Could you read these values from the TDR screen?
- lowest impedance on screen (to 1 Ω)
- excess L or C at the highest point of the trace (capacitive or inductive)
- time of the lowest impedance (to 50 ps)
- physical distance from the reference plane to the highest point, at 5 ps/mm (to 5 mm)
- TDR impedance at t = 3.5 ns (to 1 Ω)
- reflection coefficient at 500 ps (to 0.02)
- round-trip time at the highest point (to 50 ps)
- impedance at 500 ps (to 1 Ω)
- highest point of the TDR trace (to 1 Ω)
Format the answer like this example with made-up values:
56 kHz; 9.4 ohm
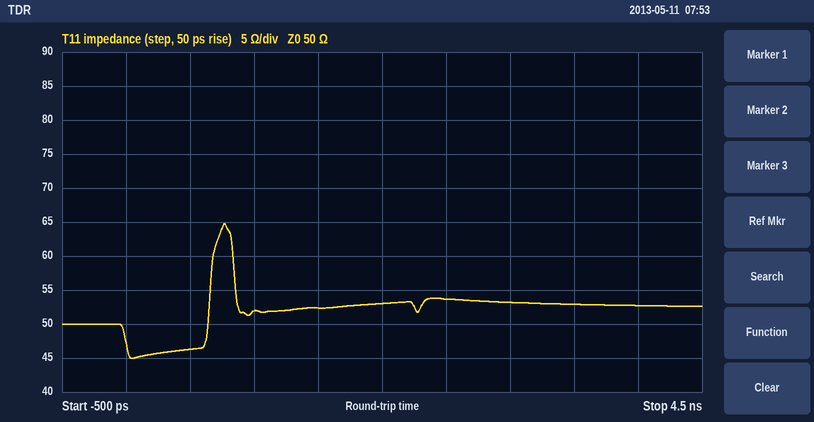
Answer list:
45 Ω; inductive; 50 ps; 75 mm; 53 Ω; -0.04; 750 ps; 46 Ω; 65 Ω
